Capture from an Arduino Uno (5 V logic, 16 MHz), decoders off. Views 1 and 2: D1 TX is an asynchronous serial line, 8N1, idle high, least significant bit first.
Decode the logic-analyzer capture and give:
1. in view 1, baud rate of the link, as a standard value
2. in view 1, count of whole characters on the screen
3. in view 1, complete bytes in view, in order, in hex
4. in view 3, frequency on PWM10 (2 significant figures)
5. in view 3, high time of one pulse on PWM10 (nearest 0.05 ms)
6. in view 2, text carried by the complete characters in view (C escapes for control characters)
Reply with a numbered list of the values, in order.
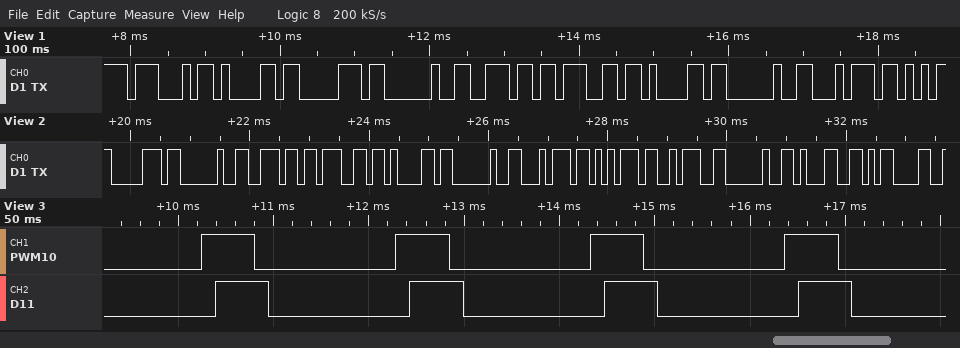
1. 9600 baud
2. 9
3. 47 61 70 20 6E 67 61 20 74
4. 490 Hz
5. 0.55 ms
6. "p nga tu: 1\r"
